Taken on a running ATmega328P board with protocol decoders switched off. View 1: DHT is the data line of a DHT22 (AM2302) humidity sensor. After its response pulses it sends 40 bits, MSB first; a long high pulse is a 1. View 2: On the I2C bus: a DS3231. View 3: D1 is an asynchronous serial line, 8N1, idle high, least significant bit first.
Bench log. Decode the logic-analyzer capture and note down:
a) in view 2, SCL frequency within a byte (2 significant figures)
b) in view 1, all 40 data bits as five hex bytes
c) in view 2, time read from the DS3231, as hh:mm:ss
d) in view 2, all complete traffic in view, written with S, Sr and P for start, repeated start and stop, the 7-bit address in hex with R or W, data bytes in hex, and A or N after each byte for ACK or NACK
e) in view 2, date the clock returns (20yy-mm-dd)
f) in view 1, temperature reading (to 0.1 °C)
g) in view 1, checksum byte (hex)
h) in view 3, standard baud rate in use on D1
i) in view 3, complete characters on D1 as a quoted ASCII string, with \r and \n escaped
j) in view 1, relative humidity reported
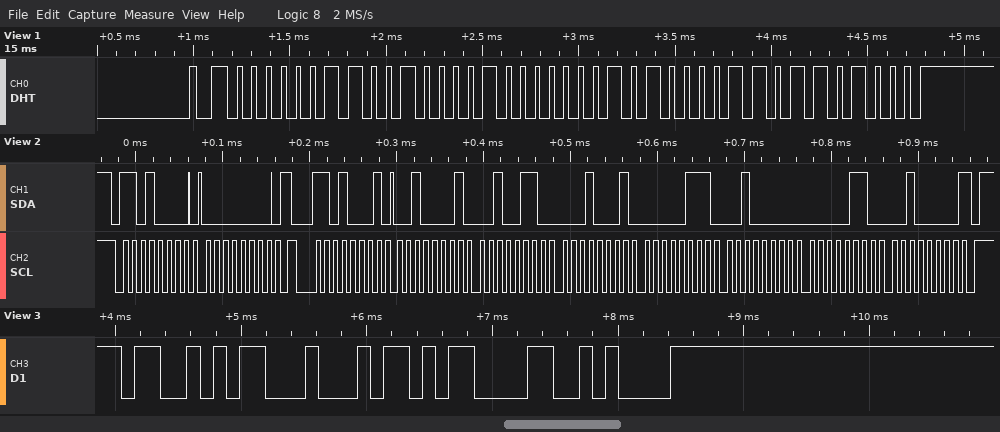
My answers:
100 kHz
03 21 01 43 68
11:26:21
S 68W A 00 A Sr 68R A 21 A 26 A 11 A 07 A 20 A 06 A 20 N P
2020-06-20
32.3 °C
0x68
9600 baud
"SD\r\n"
80.1 %
